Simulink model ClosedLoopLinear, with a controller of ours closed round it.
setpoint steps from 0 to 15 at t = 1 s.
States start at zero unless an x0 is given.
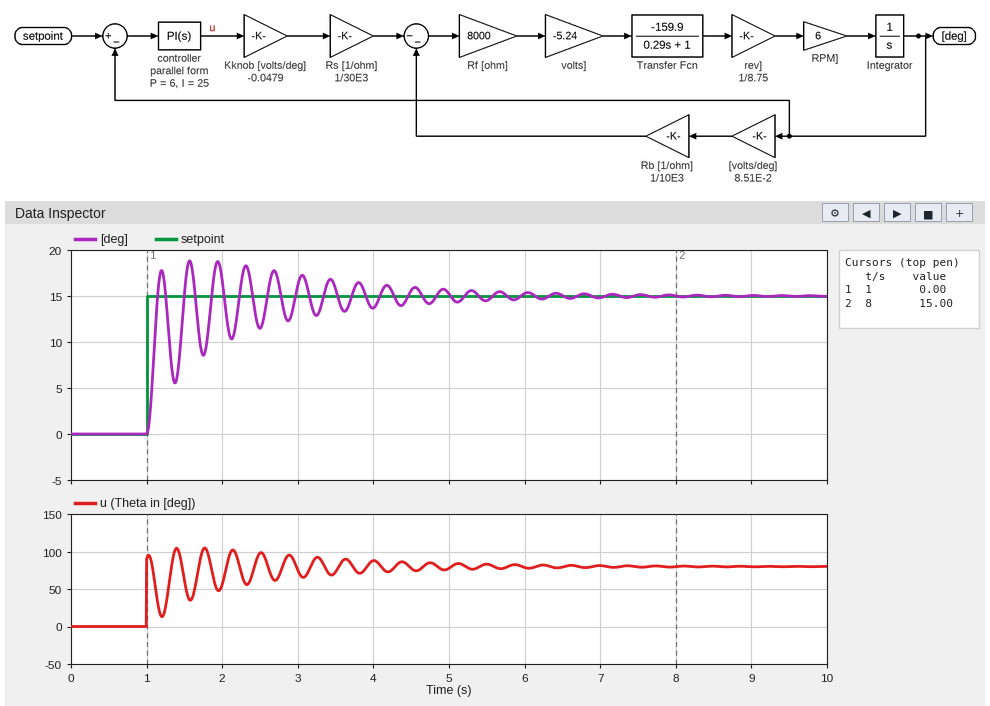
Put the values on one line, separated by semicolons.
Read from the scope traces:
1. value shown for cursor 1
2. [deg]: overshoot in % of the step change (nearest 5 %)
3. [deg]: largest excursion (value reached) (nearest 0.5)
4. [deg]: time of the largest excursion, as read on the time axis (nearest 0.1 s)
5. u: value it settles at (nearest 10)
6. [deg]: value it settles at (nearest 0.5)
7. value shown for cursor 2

0.00; 25 %; 19.0; 1.6 s; 80; 15.0; 15.00
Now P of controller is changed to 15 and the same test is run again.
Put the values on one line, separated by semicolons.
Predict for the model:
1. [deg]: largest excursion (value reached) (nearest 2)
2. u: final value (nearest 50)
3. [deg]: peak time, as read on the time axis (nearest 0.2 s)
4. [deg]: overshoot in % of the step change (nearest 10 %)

22; 100; 1.2 s; 40 %
